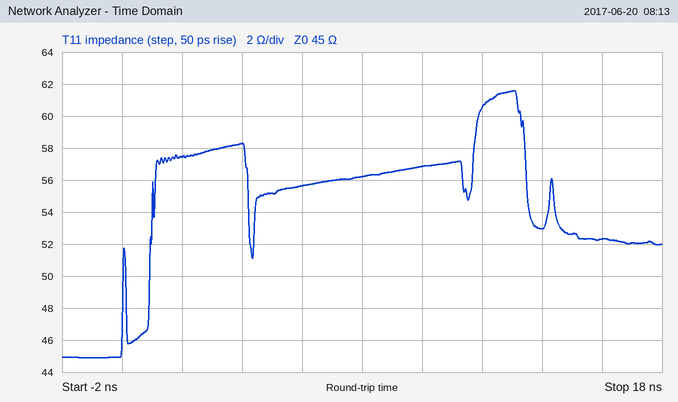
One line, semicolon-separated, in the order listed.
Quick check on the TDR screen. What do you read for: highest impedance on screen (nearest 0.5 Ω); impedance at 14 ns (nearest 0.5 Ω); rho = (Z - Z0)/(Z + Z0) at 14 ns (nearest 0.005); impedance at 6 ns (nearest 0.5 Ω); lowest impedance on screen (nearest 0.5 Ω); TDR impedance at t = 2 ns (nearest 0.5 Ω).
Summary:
61.5 Ω; 53.0 Ω; +0.080; 55.5 Ω; 45.0 Ω; 57.5 Ω
